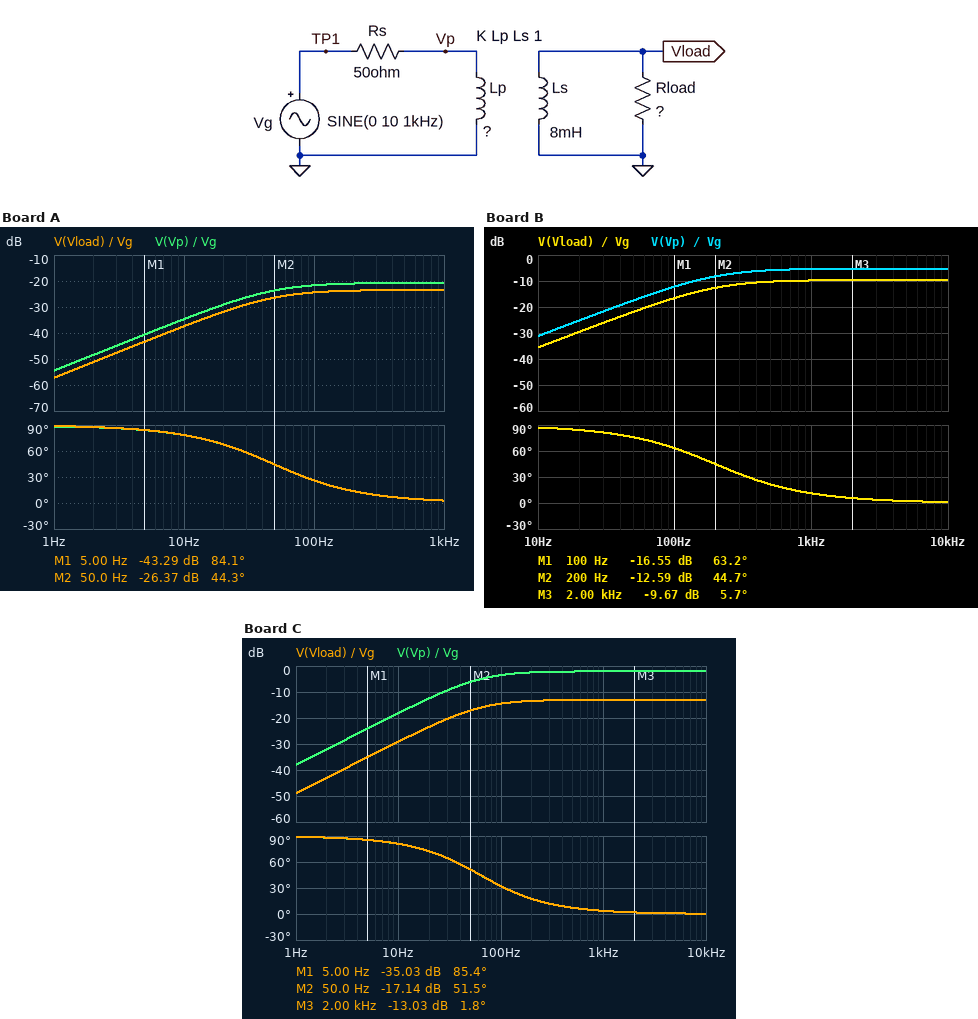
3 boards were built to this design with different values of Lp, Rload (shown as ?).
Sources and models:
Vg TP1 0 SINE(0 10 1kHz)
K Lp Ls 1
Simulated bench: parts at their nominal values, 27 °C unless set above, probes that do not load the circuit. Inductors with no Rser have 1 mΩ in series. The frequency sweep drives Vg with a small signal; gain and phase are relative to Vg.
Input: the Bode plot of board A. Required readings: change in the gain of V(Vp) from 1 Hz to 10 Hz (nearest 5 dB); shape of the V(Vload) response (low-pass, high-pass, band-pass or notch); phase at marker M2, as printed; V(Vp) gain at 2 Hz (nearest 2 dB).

20 dB
high-pass
44.3 deg
-48 dB
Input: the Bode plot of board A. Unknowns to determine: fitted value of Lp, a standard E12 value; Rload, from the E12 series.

15 mH
2.7 Ω
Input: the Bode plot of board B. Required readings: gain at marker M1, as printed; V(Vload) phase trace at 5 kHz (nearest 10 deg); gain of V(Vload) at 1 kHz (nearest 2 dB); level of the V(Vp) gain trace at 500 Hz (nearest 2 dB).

-16.55 dB
0 deg
-10 dB
-6 dB
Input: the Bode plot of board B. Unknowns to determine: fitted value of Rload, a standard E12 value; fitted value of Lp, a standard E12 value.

22 Ω
22 mH
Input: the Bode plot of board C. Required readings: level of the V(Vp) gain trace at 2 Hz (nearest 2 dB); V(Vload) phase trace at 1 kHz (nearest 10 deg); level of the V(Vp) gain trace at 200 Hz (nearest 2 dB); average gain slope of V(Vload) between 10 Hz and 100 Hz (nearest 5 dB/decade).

-32 dB
0 deg
-2 dB
15 dB/decade
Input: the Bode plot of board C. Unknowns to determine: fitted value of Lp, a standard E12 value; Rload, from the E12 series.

100 mH
15 Ω
